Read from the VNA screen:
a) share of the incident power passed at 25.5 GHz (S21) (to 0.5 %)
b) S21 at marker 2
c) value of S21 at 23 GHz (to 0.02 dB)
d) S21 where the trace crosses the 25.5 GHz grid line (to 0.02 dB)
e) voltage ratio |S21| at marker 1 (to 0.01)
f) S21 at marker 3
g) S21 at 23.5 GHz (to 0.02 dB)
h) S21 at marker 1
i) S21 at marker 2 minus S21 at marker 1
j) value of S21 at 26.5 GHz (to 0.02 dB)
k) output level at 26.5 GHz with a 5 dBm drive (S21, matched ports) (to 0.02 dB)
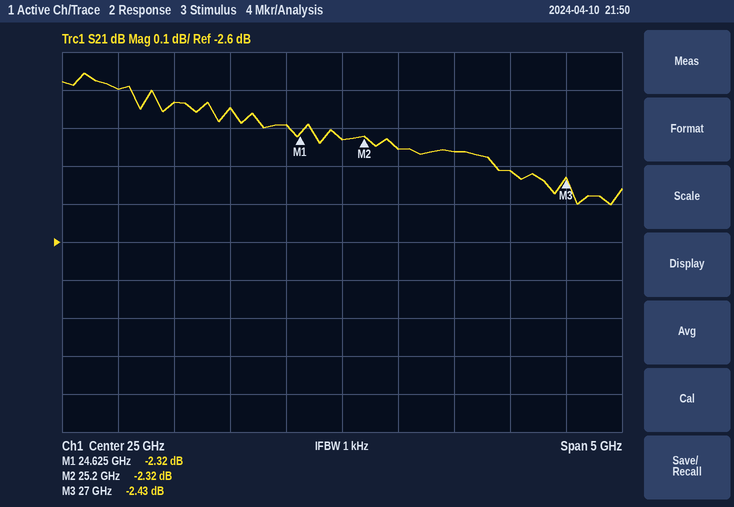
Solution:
58.0 %
-2.32 dB
-2.20 dB
-2.36 dB
0.77
-2.43 dB
-2.24 dB
-2.32 dB
0.00 dB
-2.42 dB
2.58 dBm
